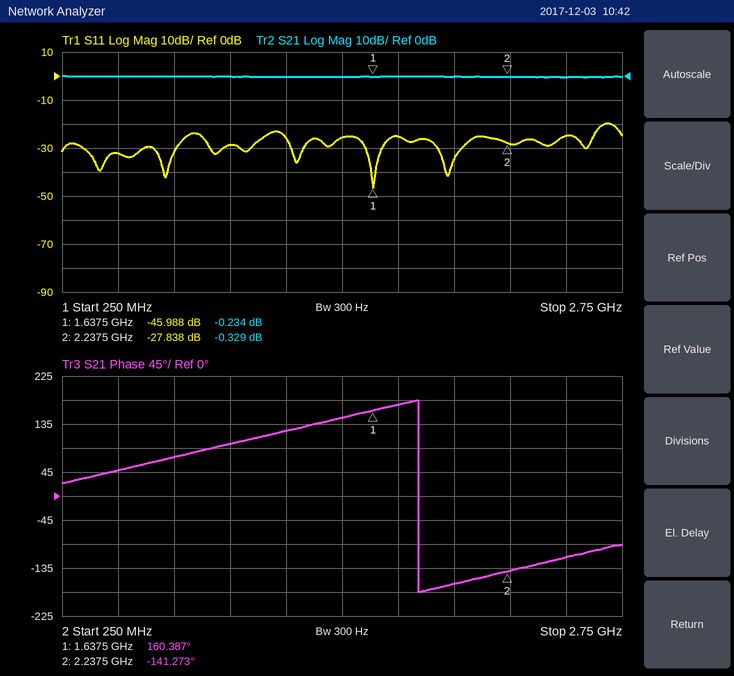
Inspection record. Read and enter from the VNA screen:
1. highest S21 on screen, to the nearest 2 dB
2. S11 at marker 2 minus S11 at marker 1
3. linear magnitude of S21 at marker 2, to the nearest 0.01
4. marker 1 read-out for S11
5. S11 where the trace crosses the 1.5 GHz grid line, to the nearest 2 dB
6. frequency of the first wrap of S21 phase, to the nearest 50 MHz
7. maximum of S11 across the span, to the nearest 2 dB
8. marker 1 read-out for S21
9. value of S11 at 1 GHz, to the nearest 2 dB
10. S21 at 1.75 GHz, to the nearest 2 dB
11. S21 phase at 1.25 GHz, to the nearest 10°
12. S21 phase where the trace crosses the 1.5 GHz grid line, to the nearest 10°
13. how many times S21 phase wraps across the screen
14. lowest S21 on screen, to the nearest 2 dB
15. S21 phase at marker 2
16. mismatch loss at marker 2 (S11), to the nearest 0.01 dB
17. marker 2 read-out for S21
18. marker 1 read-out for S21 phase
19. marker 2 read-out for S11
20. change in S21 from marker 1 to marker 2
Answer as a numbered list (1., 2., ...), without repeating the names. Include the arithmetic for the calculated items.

1. 0 dB
2. -27.838 − (-45.988) = 18.150 dB
3. 10^(-0.329/20) ≈ 0.96
4. -45.988 dB
5. -26 dB
6. 1.85 GHz
7. -20 dB
8. -0.234 dB
9. -28 dB
10. 0 dB
11. 120°
12. 150°
13. 1
14. 0 dB
15. -141.273°
16. −10 log10(1 − 10^(-27.838/10)) ≈ 0.01 dB
17. -0.329 dB
18. 160.387°
19. -27.838 dB
20. -0.329 − (-0.234) = -0.095 dB
